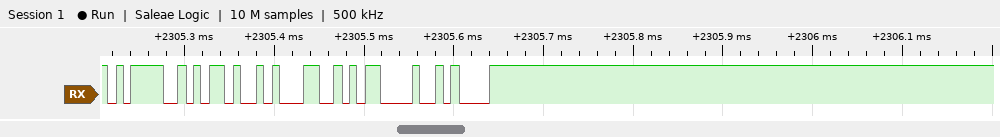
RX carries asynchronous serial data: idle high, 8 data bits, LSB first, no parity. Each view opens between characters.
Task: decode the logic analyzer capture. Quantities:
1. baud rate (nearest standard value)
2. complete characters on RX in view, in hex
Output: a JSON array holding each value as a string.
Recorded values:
["115200 baud", "3D, 2D, 31, 0D, 0A"]
